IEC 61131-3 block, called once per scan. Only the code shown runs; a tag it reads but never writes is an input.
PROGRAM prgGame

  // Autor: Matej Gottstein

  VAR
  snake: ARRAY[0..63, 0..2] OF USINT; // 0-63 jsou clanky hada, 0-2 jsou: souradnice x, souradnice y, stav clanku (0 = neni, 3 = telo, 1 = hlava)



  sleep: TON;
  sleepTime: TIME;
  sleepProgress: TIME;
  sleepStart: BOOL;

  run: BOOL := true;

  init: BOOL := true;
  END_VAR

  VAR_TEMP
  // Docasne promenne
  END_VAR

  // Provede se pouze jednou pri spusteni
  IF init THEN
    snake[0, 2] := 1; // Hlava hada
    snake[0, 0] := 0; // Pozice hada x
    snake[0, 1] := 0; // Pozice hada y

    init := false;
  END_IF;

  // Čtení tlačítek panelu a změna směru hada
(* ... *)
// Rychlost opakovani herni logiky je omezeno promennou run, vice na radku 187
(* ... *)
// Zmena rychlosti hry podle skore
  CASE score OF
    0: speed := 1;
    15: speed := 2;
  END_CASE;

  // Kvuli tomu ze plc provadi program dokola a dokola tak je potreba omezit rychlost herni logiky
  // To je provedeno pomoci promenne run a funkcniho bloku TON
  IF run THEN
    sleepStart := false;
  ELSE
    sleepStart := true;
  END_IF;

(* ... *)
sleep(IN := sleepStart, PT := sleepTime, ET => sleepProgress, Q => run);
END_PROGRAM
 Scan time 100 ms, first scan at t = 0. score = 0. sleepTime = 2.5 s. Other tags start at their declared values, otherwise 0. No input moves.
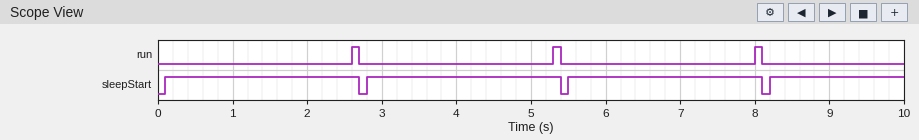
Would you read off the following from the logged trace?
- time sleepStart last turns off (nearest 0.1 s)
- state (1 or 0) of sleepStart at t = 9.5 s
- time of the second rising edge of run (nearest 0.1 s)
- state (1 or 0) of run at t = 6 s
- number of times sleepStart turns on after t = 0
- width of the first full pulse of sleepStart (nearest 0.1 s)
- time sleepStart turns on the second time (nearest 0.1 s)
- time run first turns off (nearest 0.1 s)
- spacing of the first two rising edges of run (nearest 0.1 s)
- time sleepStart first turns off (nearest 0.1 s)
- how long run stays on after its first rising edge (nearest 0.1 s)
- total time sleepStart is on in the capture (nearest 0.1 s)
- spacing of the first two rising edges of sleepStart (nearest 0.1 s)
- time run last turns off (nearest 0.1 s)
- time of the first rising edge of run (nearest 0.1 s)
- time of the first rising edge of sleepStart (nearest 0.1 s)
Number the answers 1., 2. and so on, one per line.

1. 8.1 s
2. 1
3. 5.3 s
4. 0
5. 4
6. 2.6 s
7. 2.8 s
8. 2.7 s
9. 2.7 s
10. 2.7 s
11. 0.1 s
12. 9.6 s
13. 2.7 s
14. 8.1 s
15. 2.6 s
16. 0.1 s
